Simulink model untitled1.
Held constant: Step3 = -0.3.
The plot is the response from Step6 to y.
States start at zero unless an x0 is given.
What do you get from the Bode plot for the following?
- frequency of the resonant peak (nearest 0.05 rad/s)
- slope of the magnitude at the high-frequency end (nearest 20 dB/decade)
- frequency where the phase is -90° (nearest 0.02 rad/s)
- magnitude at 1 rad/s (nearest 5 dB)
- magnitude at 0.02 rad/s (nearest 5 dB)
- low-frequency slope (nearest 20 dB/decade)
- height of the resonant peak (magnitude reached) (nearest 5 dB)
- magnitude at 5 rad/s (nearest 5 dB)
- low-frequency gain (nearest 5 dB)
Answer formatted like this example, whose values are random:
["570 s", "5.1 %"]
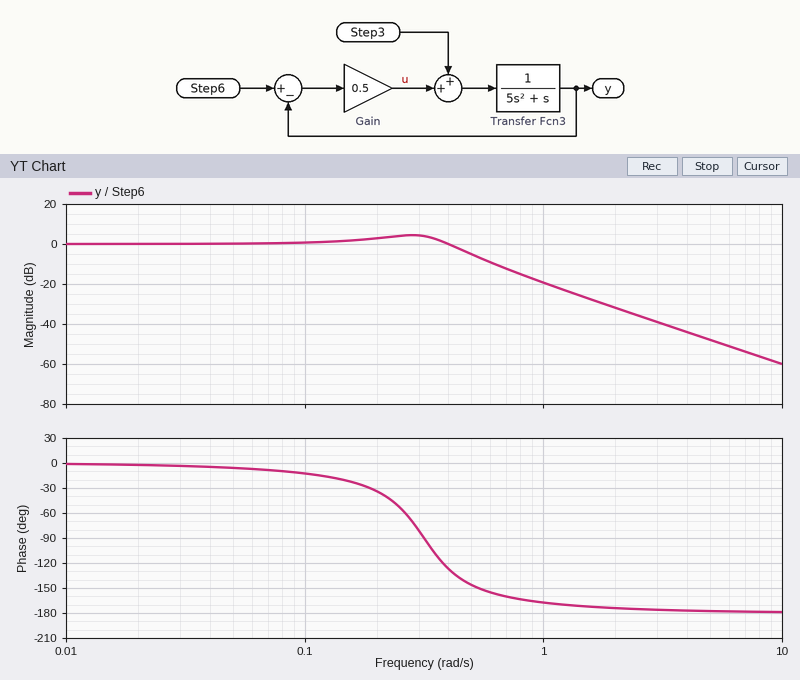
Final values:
["0.30 rad/s", "-40 dB/decade", "0.32 rad/s", "-20 dB", "0 dB", "0 dB/decade", "5 dB", "-50 dB", "0 dB"]
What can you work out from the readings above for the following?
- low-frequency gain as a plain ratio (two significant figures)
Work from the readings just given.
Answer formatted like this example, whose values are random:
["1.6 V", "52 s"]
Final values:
["1.0"]
